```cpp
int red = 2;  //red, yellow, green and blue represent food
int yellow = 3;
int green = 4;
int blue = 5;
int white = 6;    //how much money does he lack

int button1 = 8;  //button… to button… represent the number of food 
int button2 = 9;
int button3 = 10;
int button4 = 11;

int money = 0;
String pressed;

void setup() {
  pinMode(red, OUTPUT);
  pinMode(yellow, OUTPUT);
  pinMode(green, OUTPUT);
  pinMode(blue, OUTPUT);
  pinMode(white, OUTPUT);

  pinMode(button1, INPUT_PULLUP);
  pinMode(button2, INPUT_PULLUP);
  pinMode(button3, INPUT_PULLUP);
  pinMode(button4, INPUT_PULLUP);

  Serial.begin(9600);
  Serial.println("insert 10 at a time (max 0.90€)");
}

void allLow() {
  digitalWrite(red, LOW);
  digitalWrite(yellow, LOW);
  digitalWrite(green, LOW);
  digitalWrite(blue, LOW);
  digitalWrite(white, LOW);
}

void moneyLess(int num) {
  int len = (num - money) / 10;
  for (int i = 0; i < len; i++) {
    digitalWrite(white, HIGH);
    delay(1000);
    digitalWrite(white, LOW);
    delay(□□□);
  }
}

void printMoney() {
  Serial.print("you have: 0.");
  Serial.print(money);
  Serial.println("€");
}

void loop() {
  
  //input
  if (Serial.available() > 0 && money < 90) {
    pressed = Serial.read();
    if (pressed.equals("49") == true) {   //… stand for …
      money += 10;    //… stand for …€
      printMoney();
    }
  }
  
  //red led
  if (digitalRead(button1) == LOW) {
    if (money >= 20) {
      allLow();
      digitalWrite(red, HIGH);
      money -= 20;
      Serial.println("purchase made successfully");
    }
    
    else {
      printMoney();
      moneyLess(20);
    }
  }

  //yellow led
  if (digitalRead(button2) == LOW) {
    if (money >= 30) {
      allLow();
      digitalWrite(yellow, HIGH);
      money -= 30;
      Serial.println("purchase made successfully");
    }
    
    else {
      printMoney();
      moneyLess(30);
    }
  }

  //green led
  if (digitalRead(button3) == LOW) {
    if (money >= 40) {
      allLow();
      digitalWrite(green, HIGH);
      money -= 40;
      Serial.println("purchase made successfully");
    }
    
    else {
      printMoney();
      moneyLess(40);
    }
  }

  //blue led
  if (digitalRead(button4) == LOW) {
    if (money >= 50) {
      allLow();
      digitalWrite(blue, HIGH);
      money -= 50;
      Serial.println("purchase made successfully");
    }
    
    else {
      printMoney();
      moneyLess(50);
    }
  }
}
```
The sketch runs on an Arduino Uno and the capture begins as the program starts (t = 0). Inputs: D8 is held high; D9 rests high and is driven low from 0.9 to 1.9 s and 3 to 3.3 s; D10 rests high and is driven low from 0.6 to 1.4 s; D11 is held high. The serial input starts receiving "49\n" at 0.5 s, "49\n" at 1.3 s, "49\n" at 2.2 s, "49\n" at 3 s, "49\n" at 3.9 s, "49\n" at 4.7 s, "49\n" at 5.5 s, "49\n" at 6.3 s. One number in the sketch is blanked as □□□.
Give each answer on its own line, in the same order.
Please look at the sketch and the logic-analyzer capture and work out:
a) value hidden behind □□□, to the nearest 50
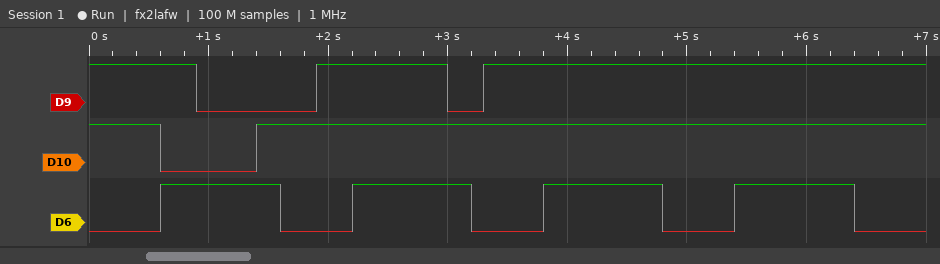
600
